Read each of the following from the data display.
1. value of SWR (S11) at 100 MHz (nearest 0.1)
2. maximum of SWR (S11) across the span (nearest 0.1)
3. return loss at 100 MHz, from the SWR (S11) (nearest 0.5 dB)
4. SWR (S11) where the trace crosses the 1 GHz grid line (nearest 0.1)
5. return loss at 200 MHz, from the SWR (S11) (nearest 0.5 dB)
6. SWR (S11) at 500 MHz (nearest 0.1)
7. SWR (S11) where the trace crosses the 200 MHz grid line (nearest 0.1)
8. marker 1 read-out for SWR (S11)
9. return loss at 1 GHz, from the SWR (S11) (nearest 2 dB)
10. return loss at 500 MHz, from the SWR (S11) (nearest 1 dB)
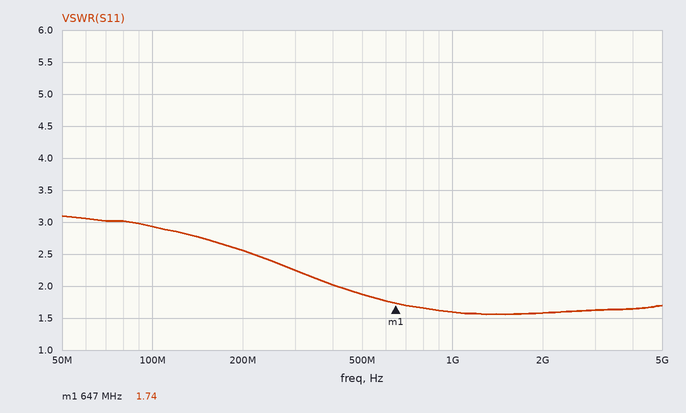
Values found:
2.9
3.1
6.0 dB
1.6
7.0 dB
1.9
2.6
1.74
12 dB
10 dB
